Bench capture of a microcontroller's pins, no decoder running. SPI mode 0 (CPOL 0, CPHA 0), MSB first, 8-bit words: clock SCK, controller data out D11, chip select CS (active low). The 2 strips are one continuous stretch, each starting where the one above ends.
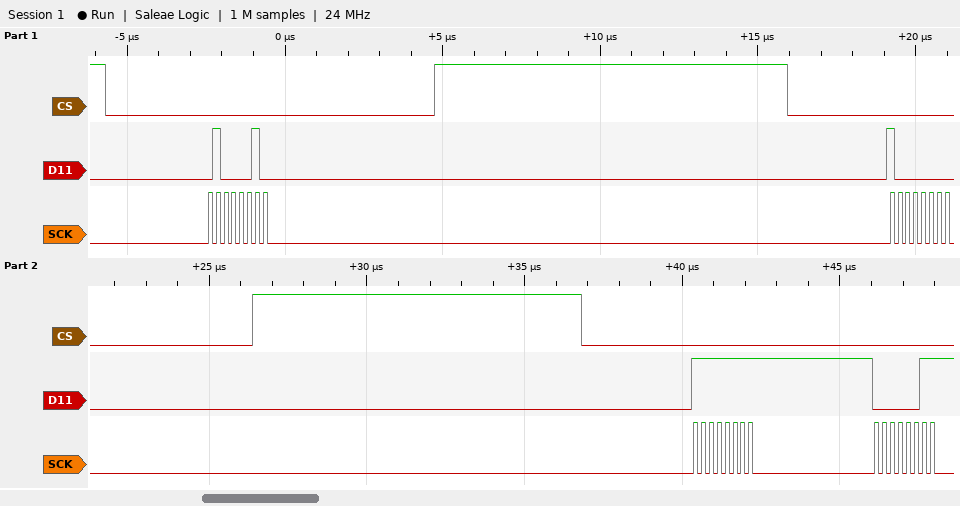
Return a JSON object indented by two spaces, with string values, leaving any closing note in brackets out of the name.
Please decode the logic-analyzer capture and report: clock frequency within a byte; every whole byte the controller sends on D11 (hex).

{
  "clock frequency within a byte": "4 MHz",
  "every whole byte the controller sends on D11": "0x42 0x80 0xFF 0x03"
}
